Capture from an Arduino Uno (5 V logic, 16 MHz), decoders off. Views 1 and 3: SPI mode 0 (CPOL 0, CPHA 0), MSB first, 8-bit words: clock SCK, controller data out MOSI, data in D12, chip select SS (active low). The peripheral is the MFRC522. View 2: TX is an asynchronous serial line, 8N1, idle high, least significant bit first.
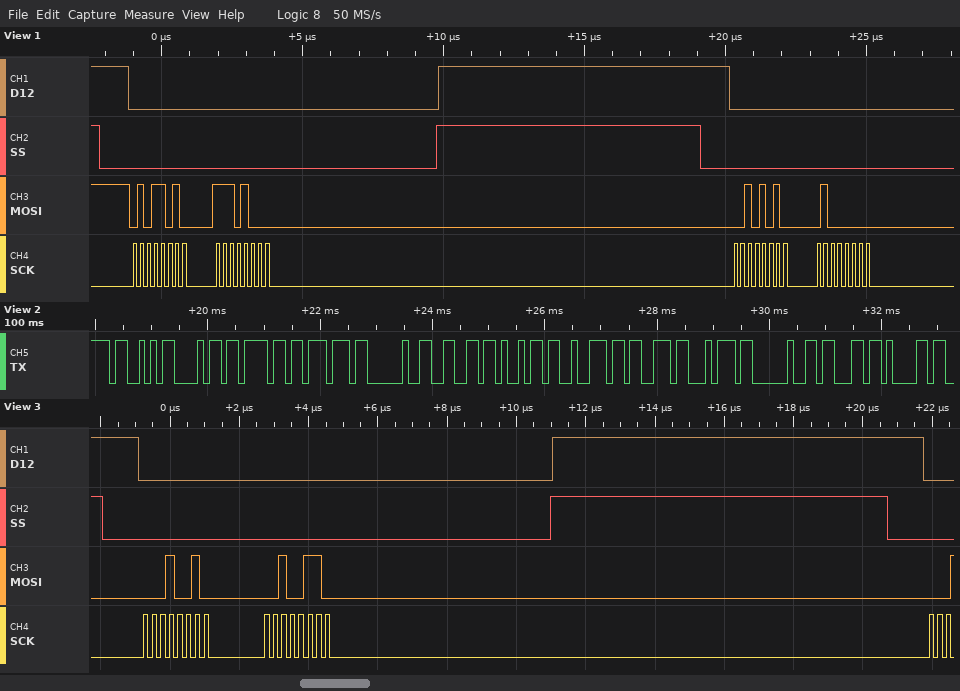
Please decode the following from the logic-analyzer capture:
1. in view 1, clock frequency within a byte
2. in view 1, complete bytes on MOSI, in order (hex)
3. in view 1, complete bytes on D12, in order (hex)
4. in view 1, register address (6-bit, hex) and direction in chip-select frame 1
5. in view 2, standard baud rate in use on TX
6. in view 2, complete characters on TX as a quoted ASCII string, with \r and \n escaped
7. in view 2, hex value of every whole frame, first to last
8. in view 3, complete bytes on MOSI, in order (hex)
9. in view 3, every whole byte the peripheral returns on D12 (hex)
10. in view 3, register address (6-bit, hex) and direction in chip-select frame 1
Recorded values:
4 MHz
5A E8 2A 40
00 00 00 00
0x2D write
9600 baud
"Show first ca"
53 68 6F 77 20 66 69 72 73 74 20 63 61
0x12 0x26
0x00 0x00
0x09 write
